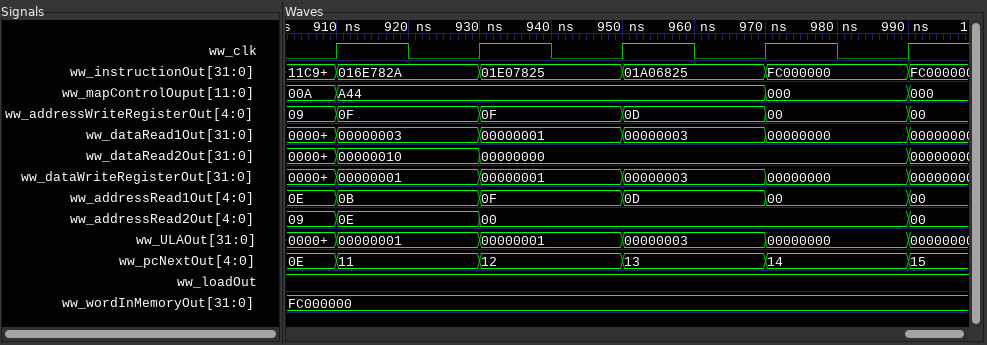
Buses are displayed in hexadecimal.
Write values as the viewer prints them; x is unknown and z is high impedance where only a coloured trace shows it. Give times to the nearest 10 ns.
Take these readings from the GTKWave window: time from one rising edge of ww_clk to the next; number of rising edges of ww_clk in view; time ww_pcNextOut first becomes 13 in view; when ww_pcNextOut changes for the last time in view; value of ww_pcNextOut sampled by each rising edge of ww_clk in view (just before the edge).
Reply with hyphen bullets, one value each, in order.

- 20 ns
- 5
- 950 ns
- 990 ns
- 0E, 11, 12, 13, 14
